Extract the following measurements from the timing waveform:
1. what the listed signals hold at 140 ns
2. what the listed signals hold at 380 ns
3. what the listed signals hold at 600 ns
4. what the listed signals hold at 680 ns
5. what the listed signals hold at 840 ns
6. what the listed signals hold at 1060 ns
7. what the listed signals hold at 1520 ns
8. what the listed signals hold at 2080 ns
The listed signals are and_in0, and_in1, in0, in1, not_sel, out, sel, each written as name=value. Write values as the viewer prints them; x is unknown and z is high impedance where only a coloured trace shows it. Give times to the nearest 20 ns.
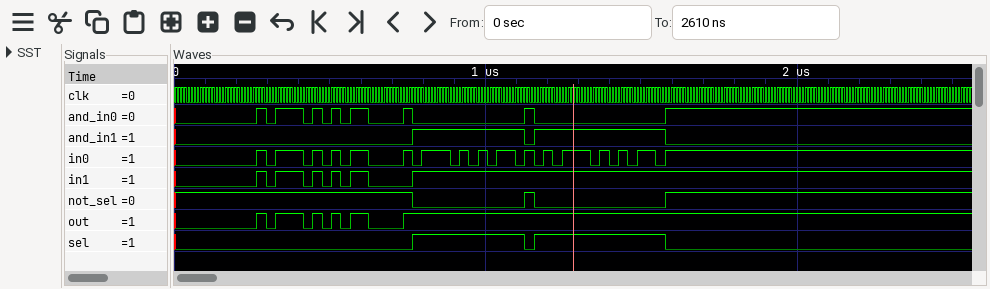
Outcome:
and_in0=0, and_in1=0, in0=0, in1=0, not_sel=1, out=0, sel=0
and_in0=1, and_in1=0, in0=1, in1=1, not_sel=1, out=1, sel=0
and_in0=1, and_in1=0, in0=1, in1=1, not_sel=1, out=1, sel=0
and_in0=0, and_in1=0, in0=0, in1=0, not_sel=1, out=0, sel=0
and_in0=0, and_in1=1, in0=1, in1=1, not_sel=0, out=1, sel=1
and_in0=0, and_in1=1, in0=1, in1=1, not_sel=0, out=1, sel=1
and_in0=0, and_in1=1, in0=1, in1=1, not_sel=0, out=1, sel=1
and_in0=1, and_in1=0, in0=1, in1=1, not_sel=1, out=1, sel=0
